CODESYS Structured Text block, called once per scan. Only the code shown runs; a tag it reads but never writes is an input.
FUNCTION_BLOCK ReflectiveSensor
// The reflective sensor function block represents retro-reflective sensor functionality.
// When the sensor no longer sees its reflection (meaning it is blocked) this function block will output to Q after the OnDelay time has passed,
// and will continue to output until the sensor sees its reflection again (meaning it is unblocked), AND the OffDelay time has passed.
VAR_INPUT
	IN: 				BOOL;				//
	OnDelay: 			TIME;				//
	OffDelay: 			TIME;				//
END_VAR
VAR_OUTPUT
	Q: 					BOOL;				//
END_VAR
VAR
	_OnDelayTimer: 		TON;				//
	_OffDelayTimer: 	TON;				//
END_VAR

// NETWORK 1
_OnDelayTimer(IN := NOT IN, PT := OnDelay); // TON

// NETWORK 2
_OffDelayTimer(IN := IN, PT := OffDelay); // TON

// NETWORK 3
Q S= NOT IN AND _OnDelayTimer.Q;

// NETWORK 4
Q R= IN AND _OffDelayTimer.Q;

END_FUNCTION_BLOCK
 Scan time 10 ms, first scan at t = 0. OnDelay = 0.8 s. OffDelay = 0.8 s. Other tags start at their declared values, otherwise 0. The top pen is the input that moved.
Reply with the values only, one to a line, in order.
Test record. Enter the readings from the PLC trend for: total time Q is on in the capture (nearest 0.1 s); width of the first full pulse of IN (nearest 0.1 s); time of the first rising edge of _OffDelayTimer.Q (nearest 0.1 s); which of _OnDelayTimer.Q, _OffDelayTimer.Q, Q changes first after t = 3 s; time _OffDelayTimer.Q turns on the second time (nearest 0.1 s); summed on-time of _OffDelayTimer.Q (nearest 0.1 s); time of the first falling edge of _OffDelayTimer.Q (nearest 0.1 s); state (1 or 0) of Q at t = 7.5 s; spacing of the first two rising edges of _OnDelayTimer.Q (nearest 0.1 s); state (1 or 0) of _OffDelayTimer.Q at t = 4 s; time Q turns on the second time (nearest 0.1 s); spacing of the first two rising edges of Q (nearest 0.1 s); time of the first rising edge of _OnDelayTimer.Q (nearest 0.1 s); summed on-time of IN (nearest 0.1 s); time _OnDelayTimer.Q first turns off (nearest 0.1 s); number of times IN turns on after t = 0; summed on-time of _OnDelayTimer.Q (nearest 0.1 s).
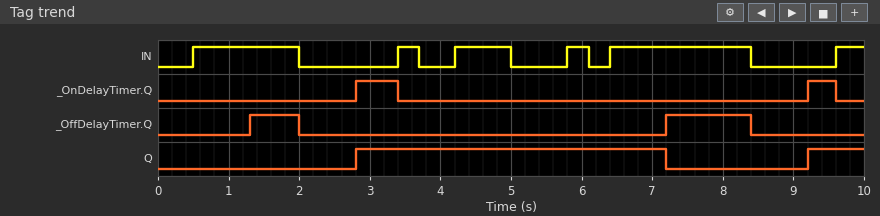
5.2 s
1.5 s
1.3 s
_OnDelayTimer.Q
7.2 s
1.9 s
2.0 s
0
6.4 s
0
9.2 s
6.4 s
2.8 s
5.3 s
3.4 s
6
1.0 s
